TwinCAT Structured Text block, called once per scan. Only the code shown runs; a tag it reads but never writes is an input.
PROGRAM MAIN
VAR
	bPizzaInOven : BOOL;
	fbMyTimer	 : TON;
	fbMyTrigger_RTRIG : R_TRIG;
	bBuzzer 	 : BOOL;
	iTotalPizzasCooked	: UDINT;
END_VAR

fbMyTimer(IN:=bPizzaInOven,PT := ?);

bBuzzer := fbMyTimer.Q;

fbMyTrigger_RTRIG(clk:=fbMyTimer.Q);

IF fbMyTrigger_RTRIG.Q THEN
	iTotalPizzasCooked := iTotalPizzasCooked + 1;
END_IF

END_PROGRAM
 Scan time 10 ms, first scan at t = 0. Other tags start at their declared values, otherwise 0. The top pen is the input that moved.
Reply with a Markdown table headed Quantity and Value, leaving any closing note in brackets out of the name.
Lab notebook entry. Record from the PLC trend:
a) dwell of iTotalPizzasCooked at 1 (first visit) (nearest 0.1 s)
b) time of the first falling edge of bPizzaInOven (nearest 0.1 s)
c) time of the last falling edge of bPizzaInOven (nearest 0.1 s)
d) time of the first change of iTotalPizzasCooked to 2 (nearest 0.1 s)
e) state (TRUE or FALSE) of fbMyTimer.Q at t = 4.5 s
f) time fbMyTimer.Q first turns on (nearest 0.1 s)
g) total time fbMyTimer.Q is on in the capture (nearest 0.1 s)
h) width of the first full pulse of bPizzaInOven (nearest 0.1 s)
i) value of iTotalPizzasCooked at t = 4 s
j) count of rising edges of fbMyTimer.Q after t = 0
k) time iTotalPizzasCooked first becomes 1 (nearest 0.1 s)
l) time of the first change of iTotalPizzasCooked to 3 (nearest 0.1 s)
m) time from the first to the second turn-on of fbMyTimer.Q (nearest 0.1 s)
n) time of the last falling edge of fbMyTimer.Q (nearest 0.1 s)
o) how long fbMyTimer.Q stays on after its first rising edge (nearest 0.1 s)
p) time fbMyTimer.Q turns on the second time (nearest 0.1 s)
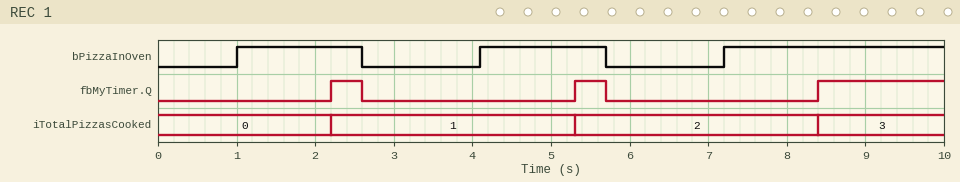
| Quantity | Value |
|---|---|
| dwell of iTotalPizzasCooked at 1 (first visit) | 3.1 s |
| time of the first falling edge of bPizzaInOven | 2.6 s |
| time of the last falling edge of bPizzaInOven | 5.7 s |
| time of the first change of iTotalPizzasCooked to 2 | 5.3 s |
| state (TRUE or FALSE) of fbMyTimer.Q at t = 4.5 s | FALSE |
| time fbMyTimer.Q first turns on | 2.2 s |
| total time fbMyTimer.Q is on in the capture | 2.4 s |
| width of the first full pulse of bPizzaInOven | 1.6 s |
| value of iTotalPizzasCooked at t = 4 s | 1 |
| count of rising edges of fbMyTimer.Q after t = 0 | 3 |
| time iTotalPizzasCooked first becomes 1 | 2.2 s |
| time of the first change of iTotalPizzasCooked to 3 | 8.4 s |
| time from the first to the second turn-on of fbMyTimer.Q | 3.1 s |
| time of the last falling edge of fbMyTimer.Q | 5.7 s |
| how long fbMyTimer.Q stays on after its first rising edge | 0.4 s |
| time fbMyTimer.Q turns on the second time | 5.3 s |
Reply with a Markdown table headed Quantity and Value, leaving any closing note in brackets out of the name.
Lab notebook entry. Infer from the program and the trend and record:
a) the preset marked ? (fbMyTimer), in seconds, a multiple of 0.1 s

| Quantity | Value |
|---|---|
| the preset marked ? (fbMyTimer), in seconds, a multiple of 0.1 s | 1.2 s |
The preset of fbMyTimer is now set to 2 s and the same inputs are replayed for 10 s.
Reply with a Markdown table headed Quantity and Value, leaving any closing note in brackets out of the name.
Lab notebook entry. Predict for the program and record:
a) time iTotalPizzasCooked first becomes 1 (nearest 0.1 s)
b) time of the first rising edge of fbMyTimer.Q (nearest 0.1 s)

| Quantity | Value |
|---|---|
| time iTotalPizzasCooked first becomes 1 | 9.2 s |
| time of the first rising edge of fbMyTimer.Q | 9.2 s |
